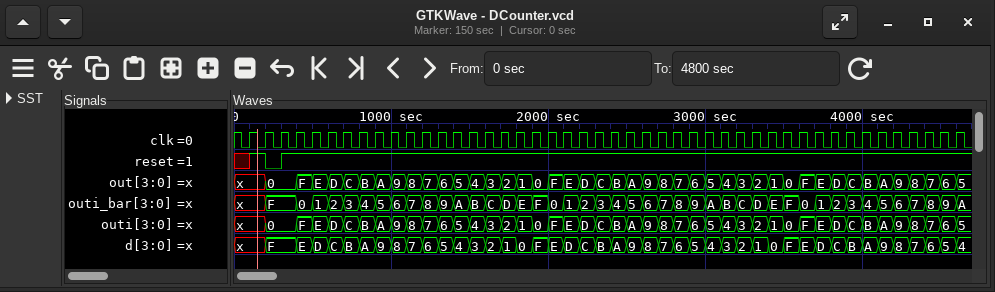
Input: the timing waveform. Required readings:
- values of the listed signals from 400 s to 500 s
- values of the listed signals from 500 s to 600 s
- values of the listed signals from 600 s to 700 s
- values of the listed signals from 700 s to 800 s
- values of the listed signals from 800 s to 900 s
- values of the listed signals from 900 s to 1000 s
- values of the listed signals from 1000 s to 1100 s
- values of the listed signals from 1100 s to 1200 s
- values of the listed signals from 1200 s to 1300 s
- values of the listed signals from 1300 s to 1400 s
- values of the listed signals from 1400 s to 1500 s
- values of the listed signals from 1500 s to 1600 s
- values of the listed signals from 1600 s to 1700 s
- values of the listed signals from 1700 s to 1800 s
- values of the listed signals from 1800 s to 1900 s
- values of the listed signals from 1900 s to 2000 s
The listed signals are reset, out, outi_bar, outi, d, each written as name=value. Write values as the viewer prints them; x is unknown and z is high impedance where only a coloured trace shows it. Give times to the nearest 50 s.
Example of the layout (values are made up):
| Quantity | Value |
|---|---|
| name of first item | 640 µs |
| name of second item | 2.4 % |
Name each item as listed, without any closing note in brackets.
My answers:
| Quantity | Value |
|---|---|
| values of the listed signals from 400 s to 500 s | reset=1, out=F, outi_bar=0, outi=F, d=E |
| values of the listed signals from 500 s to 600 s | reset=1, out=E, outi_bar=1, outi=E, d=D |
| values of the listed signals from 600 s to 700 s | reset=1, out=D, outi_bar=2, outi=D, d=C |
| values of the listed signals from 700 s to 800 s | reset=1, out=C, outi_bar=3, outi=C, d=B |
| values of the listed signals from 800 s to 900 s | reset=1, out=B, outi_bar=4, outi=B, d=A |
| values of the listed signals from 900 s to 1000 s | reset=1, out=A, outi_bar=5, outi=A, d=9 |
| values of the listed signals from 1000 s to 1100 s | reset=1, out=9, outi_bar=6, outi=9, d=8 |
| values of the listed signals from 1100 s to 1200 s | reset=1, out=8, outi_bar=7, outi=8, d=7 |
| values of the listed signals from 1200 s to 1300 s | reset=1, out=7, outi_bar=8, outi=7, d=6 |
| values of the listed signals from 1300 s to 1400 s | reset=1, out=6, outi_bar=9, outi=6, d=5 |
| values of the listed signals from 1400 s to 1500 s | reset=1, out=5, outi_bar=A, outi=5, d=4 |
| values of the listed signals from 1500 s to 1600 s | reset=1, out=4, outi_bar=B, outi=4, d=3 |
| values of the listed signals from 1600 s to 1700 s | reset=1, out=3, outi_bar=C, outi=3, d=2 |
| values of the listed signals from 1700 s to 1800 s | reset=1, out=2, outi_bar=D, outi=2, d=1 |
| values of the listed signals from 1800 s to 1900 s | reset=1, out=1, outi_bar=E, outi=1, d=0 |
| values of the listed signals from 1900 s to 2000 s | reset=1, out=0, outi_bar=F, outi=0, d=F |
